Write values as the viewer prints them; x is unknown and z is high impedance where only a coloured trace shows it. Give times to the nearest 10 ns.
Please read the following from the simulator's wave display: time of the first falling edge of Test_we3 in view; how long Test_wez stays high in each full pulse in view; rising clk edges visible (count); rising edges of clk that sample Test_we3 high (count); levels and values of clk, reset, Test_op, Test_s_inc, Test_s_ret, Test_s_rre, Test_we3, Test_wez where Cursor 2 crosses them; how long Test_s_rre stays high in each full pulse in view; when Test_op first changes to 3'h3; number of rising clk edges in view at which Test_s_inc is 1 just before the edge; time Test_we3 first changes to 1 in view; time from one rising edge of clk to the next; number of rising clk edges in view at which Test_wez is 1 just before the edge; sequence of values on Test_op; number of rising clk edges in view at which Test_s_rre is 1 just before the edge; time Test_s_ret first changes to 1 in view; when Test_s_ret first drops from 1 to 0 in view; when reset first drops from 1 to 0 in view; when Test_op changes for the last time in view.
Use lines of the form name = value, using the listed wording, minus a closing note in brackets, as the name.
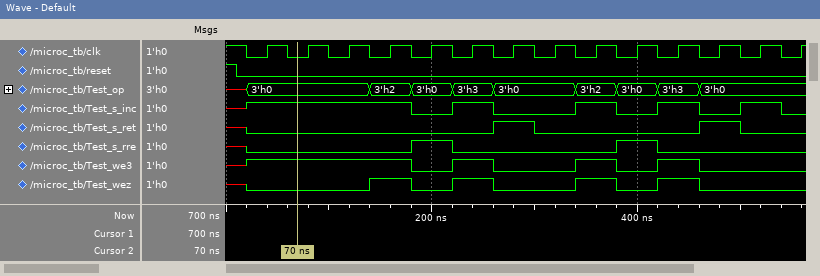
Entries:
time of the first falling edge of Test_we3 in view = 180 ns
how long Test_wez stays high in each full pulse in view = 40 ns, 40 ns, 40 ns, 40 ns
rising clk edges visible = 14
rising edges of clk that sample Test_we3 high = 7
levels and values of clk, reset, Test_op, Test_s_inc, Test_s_ret, Test_s_rre, Test_we3, Test_wez where Cursor 2 crosses them = clk=0, reset=0, Test_op=3'h0, Test_s_inc=1, Test_s_ret=0, Test_s_rre=0, Test_we3=1, Test_wez=0
how long Test_s_rre stays high in each full pulse in view = 40 ns, 40 ns
when Test_op first changes to 3'h3 = 220 ns
number of rising clk edges in view at which Test_s_inc is 1 just before the edge = 8
time Test_we3 first changes to 1 in view = 20 ns
time from one rising edge of clk to the next = 40 ns
number of rising clk edges in view at which Test_wez is 1 just before the edge = 4
sequence of values on Test_op = x, 3'h0, 3'h2, 3'h0, 3'h3, 3'h0, 3'h2, 3'h0, 3'h3, 3'h0
number of rising clk edges in view at which Test_s_rre is 1 just before the edge = 2
time Test_s_ret first changes to 1 in view = 260 ns
when Test_s_ret first drops from 1 to 0 in view = 300 ns
when reset first drops from 1 to 0 in view = 10 ns
when Test_op changes for the last time in view = 460 ns
